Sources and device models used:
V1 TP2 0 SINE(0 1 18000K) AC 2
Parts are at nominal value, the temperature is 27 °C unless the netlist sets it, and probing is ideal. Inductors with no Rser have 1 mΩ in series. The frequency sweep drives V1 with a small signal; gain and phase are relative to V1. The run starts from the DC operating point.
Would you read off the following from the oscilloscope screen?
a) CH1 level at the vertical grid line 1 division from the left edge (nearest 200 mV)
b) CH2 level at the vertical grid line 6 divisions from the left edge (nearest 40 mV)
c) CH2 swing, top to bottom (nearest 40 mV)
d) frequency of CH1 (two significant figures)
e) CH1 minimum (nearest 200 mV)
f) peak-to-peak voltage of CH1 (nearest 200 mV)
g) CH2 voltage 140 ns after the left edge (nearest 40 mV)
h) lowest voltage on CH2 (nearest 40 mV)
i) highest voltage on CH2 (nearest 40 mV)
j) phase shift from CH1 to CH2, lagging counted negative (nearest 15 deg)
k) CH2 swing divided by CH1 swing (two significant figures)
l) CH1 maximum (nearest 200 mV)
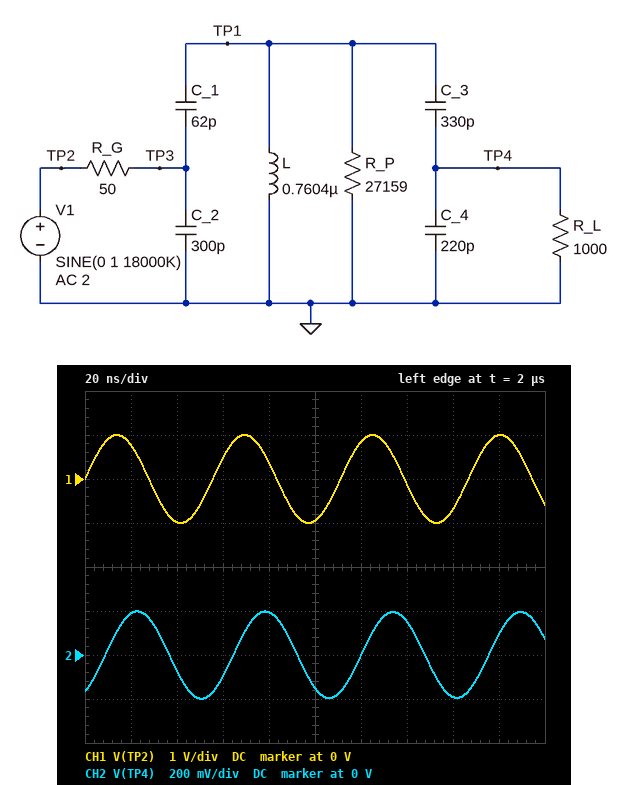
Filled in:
800 mV
0 V
400 mV
18 MHz
-1.0 V
2.0 V
160 mV
-200 mV
200 mV
-60 deg
0.20
1.0 V
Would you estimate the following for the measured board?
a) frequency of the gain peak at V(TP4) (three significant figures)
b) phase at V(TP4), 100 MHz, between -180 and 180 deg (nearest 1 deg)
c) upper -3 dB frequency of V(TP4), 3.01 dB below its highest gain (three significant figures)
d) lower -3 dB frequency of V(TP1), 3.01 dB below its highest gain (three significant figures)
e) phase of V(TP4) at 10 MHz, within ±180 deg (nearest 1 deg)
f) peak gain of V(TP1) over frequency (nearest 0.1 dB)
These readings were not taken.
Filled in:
13.4 MHz
-84 deg
13.7 MHz
13.0 MHz
128 deg
11.0 dB
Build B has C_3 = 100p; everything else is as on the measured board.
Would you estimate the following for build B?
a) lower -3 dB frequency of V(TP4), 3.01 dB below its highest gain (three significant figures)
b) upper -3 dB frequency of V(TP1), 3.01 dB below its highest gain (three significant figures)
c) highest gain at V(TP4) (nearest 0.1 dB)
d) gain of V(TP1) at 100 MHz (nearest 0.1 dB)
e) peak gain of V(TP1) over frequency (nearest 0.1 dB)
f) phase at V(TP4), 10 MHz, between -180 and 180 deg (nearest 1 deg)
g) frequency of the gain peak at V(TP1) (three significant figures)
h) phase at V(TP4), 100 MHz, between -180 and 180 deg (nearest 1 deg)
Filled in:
16.1 MHz
16.9 MHz
4.1 dB
-26.7 dB
14.2 dB
132 deg
16.5 MHz
-84 deg
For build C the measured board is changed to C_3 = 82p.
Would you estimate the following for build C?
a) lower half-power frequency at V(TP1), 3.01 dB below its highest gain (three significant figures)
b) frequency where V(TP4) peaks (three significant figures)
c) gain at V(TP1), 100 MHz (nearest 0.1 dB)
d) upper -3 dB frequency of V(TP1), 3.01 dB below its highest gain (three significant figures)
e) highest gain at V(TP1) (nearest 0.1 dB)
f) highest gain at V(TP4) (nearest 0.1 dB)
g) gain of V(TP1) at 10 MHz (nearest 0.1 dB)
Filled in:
16.7 MHz
17.1 MHz
-26.0 dB
17.6 MHz
14.5 dB
3.2 dB
-14.5 dB
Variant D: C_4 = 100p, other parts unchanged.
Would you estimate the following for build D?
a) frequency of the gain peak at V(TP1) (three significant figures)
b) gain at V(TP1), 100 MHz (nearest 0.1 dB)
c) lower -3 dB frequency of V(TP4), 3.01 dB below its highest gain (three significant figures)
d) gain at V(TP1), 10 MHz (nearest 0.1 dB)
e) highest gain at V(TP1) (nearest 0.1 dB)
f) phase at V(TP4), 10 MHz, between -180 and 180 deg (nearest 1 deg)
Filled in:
16.0 MHz
-27.2 dB
15.3 MHz
-13.8 dB
8.9 dB
129 deg
